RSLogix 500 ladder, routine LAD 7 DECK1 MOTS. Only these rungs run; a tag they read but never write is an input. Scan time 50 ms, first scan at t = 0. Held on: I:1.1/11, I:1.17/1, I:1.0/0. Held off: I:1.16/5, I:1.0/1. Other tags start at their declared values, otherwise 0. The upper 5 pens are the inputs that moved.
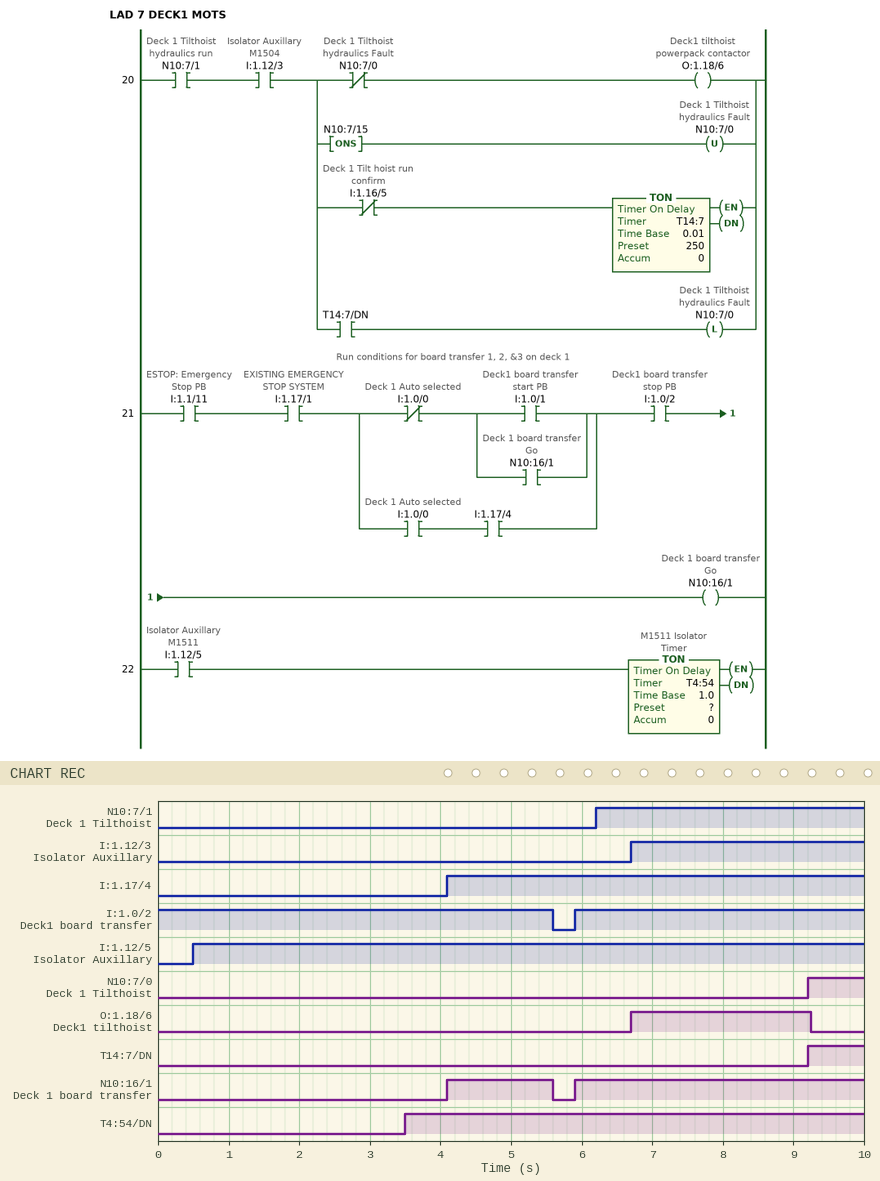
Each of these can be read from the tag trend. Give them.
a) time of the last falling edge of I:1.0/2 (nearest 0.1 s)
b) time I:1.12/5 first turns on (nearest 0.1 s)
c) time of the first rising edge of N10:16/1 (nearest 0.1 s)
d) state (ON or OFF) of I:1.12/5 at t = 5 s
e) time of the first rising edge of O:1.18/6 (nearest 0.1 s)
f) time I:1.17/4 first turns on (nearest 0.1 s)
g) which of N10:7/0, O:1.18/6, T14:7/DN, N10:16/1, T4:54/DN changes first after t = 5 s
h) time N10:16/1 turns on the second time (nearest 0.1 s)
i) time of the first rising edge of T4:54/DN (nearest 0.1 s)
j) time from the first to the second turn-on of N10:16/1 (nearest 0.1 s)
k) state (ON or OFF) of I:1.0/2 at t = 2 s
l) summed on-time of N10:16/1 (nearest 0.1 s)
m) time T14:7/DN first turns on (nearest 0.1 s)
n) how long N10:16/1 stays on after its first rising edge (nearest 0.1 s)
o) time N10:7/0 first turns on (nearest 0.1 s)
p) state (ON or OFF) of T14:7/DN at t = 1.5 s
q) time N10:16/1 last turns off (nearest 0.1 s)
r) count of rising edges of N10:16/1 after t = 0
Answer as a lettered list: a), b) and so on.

a) 5.6 s
b) 0.5 s
c) 4.1 s
d) ON
e) 6.7 s
f) 4.1 s
g) N10:16/1
h) 5.9 s
i) 3.5 s
j) 1.8 s
k) ON
l) 5.6 s
m) 9.2 s
n) 1.5 s
o) 9.2 s
p) OFF
q) 5.6 s
r) 2
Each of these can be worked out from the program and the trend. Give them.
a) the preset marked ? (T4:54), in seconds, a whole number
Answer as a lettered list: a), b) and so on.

a) 3 s
